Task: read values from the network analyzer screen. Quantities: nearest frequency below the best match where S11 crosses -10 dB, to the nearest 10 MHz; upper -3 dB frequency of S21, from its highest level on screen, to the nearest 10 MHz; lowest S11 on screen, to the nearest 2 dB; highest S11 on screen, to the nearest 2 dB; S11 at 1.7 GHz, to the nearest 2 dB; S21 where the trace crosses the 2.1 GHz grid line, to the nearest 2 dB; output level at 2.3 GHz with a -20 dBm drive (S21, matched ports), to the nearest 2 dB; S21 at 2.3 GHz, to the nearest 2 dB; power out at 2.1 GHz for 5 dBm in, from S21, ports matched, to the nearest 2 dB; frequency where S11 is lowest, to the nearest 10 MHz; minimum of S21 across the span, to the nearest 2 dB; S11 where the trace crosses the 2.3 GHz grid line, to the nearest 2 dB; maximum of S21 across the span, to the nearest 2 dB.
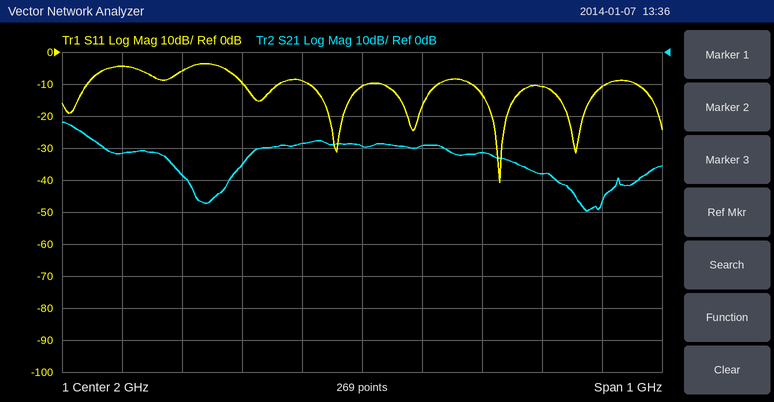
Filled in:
2.18 GHz
1.53 GHz
-40 dB
-4 dB
-6 dB
-30 dB
-58 dBm
-38 dB
-24 dBm
2.23 GHz
-50 dB
-10 dB
-22 dB
